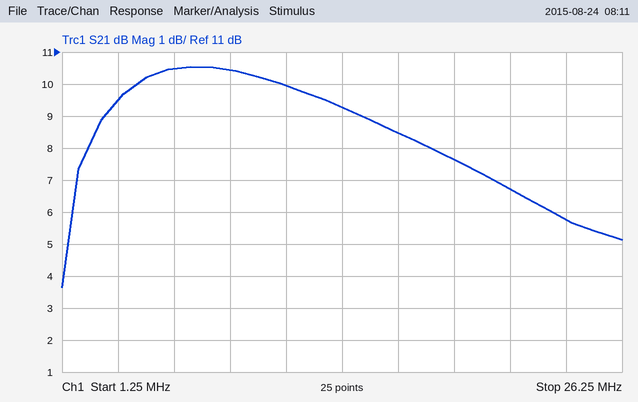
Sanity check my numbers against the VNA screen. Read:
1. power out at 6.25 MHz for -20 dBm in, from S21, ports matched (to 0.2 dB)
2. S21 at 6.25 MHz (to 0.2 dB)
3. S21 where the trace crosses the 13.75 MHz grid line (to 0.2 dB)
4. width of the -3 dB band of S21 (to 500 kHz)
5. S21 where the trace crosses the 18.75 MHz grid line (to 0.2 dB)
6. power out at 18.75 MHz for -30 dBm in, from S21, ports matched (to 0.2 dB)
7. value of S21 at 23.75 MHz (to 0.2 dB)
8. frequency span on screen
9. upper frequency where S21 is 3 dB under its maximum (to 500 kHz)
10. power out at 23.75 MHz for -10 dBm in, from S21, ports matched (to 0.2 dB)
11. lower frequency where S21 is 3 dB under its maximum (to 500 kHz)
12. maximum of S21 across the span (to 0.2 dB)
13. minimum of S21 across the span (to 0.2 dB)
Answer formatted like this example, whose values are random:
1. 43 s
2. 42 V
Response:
1. -9.6 dBm
2. 10.4 dB
3. 9.2 dB
4. 17.0 MHz
5. 7.6 dB
6. -22.4 dBm
7. 5.8 dB
8. 25 MHz
9. 19.0 MHz
10. -4.2 dBm
11. 2.0 MHz
12. 10.6 dB
13. 3.6 dB
